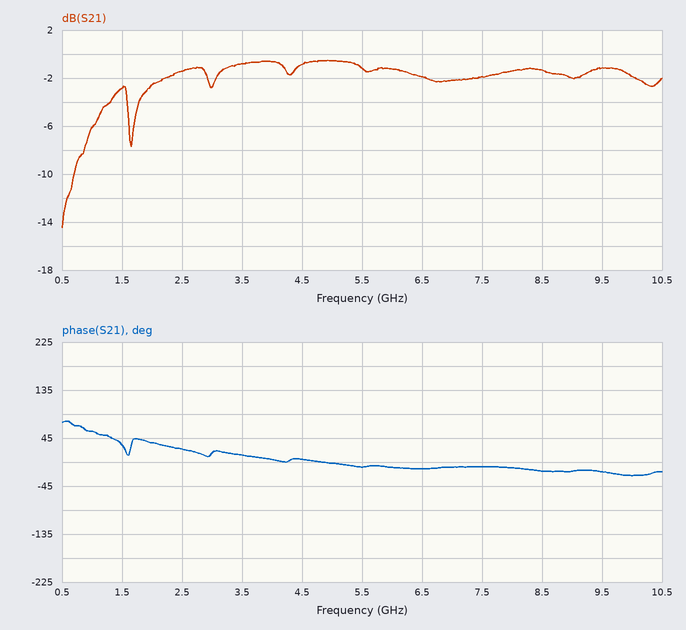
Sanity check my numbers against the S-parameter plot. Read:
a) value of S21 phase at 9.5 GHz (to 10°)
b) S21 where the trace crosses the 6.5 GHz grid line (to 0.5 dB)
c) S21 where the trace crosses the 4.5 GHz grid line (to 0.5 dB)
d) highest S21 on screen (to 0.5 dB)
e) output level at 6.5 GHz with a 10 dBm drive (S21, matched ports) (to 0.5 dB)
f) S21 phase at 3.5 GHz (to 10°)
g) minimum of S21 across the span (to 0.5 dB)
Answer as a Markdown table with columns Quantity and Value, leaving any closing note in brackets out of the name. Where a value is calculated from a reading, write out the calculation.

| Quantity | Value |
|---|---|
| value of S21 phase at 9.5 GHz | -20° |
| S21 where the trace crosses the 6.5 GHz grid line | -2.0 dB |
| S21 where the trace crosses the 4.5 GHz grid line | -1.0 dB |
| highest S21 on screen | -0.5 dB |
| output level at 6.5 GHz with a 10 dBm drive (S21, matched ports) | 10 dBm + (-2.0 dB) = 8.0 dBm |
| S21 phase at 3.5 GHz | 10° |
| minimum of S21 across the span | -14.5 dB |
